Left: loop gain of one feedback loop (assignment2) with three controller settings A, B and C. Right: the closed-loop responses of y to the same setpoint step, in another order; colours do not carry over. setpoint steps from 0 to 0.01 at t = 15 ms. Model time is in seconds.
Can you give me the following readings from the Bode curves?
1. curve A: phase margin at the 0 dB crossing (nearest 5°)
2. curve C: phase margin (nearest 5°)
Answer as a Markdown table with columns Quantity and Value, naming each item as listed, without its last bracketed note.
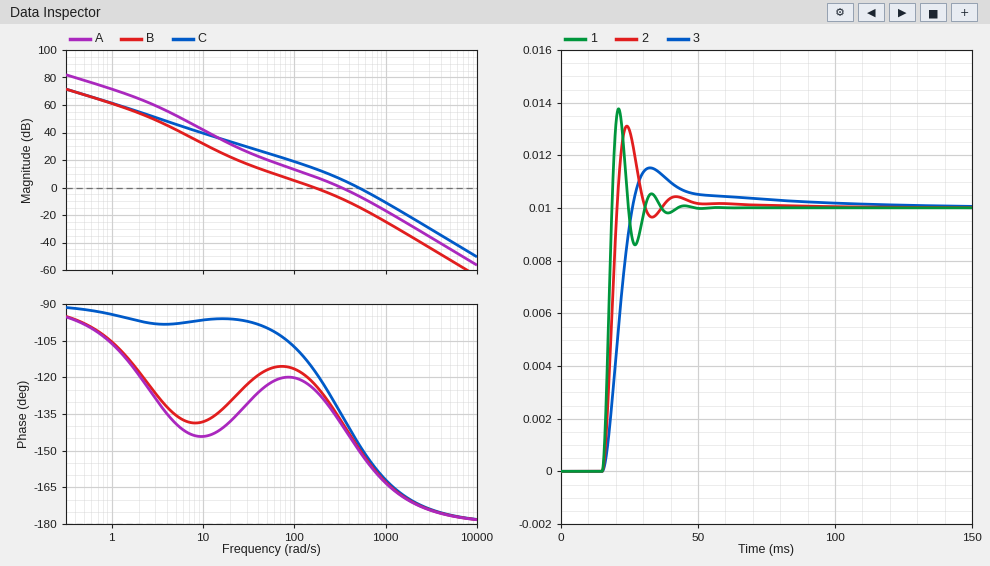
| Quantity | Value |
|---|---|
| curve A: phase margin at the 0 dB crossing | 40° |
| curve C: phase margin | 35° |
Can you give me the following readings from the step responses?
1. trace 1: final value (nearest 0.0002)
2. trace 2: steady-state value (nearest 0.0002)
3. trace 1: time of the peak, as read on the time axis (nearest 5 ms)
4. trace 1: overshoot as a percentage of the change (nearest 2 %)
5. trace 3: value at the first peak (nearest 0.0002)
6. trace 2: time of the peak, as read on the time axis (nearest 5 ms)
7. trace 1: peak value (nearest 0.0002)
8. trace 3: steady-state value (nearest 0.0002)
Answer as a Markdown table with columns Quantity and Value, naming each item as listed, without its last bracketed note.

| Quantity | Value |
|---|---|
| trace 1: final value | 0.0100 |
| trace 2: steady-state value | 0.0100 |
| trace 1: time of the peak, as read on the time axis | 20 ms |
| trace 1: overshoot as a percentage of the change | 38 % |
| trace 3: value at the first peak | 0.0116 |
| trace 2: time of the peak, as read on the time axis | 25 ms |
| trace 1: peak value | 0.0138 |
| trace 3: steady-state value | 0.0100 |
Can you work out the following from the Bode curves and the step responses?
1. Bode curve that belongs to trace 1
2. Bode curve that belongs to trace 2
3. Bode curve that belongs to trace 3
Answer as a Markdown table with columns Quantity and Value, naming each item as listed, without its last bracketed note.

| Quantity | Value |
|---|---|
| Bode curve that belongs to trace 1 | C |
| Bode curve that belongs to trace 2 | A |
| Bode curve that belongs to trace 3 | B |
